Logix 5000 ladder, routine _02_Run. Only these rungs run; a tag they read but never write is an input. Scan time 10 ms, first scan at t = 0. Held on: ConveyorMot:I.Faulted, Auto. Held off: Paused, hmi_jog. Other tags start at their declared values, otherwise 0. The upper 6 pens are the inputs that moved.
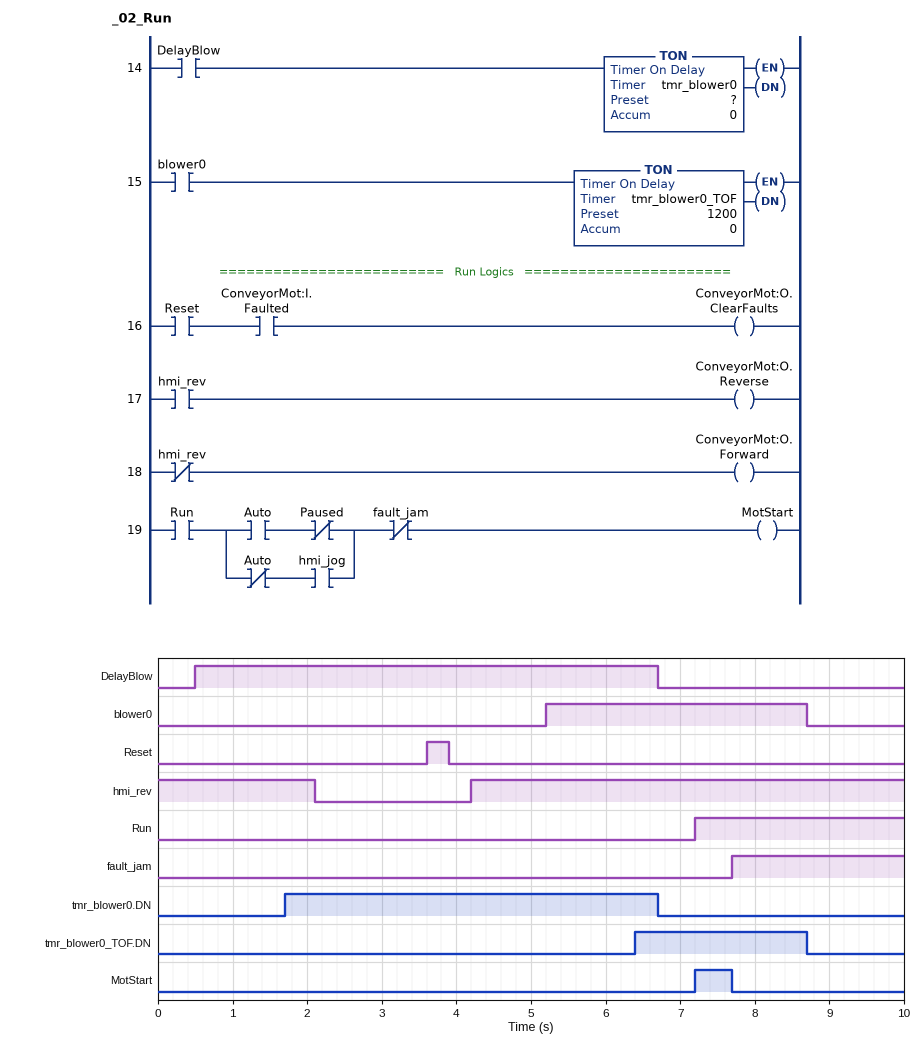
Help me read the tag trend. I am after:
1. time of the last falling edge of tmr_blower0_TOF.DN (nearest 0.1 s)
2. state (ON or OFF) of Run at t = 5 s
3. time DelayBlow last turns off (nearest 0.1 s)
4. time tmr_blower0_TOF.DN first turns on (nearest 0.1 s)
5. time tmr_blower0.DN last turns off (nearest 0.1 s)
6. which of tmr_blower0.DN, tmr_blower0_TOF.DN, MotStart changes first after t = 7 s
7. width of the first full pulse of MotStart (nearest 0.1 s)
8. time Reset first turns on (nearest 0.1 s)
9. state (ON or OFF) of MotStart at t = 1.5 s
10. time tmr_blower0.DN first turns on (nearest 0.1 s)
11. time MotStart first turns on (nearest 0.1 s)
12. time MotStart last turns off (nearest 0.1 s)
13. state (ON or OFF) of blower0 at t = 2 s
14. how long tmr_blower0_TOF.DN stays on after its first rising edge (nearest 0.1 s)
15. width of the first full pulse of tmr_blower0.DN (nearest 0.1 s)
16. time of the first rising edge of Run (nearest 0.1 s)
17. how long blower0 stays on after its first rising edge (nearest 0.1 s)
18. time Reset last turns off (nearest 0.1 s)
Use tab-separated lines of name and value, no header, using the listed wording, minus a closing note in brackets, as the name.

time of the last falling edge of tmr_blower0_TOF.DN	8.7 s
state (ON or OFF) of Run at t = 5 s	OFF
time DelayBlow last turns off	6.7 s
time tmr_blower0_TOF.DN first turns on	6.4 s
time tmr_blower0.DN last turns off	6.7 s
which of tmr_blower0.DN, tmr_blower0_TOF.DN, MotStart changes first after t = 7 s	MotStart
width of the first full pulse of MotStart	0.5 s
time Reset first turns on	3.6 s
state (ON or OFF) of MotStart at t = 1.5 s	OFF
time tmr_blower0.DN first turns on	1.7 s
time MotStart first turns on	7.2 s
time MotStart last turns off	7.7 s
state (ON or OFF) of blower0 at t = 2 s	OFF
how long tmr_blower0_TOF.DN stays on after its first rising edge	2.3 s
width of the first full pulse of tmr_blower0.DN	5.0 s
time of the first rising edge of Run	7.2 s
how long blower0 stays on after its first rising edge	3.5 s
time Reset last turns off	3.9 s
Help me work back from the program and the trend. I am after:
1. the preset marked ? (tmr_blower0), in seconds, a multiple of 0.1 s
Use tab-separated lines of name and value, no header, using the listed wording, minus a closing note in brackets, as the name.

the preset marked ? (tmr_blower0), in seconds, a multiple of 0.1 s	1.2 s
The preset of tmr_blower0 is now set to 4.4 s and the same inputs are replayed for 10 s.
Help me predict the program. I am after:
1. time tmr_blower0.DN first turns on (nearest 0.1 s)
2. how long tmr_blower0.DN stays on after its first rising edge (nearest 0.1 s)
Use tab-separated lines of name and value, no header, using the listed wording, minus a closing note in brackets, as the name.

time tmr_blower0.DN first turns on	4.9 s
how long tmr_blower0.DN stays on after its first rising edge	1.8 s
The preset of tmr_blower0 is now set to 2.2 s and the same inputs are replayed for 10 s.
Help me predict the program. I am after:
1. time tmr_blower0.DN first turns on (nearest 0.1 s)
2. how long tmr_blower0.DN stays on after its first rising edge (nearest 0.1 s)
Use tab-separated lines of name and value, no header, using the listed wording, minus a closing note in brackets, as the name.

time tmr_blower0.DN first turns on	2.7 s
how long tmr_blower0.DN stays on after its first rising edge	4.0 s
